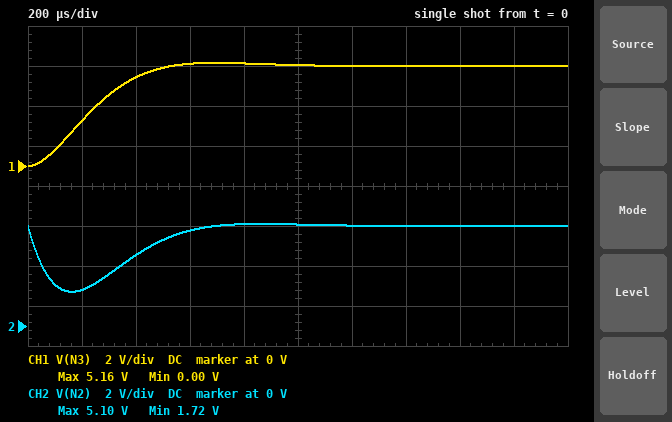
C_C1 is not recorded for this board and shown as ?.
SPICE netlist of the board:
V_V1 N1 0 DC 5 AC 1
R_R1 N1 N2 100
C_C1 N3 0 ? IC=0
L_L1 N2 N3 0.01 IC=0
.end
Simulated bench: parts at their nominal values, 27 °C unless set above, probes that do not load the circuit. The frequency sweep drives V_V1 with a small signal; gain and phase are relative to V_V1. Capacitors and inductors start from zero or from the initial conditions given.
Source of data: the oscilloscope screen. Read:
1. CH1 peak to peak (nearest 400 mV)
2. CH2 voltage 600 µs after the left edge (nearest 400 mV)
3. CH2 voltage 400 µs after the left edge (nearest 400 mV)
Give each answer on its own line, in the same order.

5.2 V
4.8 V
3.6 V
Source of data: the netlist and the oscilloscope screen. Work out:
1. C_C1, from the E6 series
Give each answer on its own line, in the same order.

2.2 µF
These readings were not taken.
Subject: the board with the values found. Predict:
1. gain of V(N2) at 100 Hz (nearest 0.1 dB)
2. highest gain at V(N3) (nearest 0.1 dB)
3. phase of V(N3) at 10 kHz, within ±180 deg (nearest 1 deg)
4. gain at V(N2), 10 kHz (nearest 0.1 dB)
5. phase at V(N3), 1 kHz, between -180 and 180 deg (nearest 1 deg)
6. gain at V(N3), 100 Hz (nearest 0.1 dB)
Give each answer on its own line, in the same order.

-0.1 dB
0 dB
-171 deg
-0.1 dB
-85 deg
0 dB
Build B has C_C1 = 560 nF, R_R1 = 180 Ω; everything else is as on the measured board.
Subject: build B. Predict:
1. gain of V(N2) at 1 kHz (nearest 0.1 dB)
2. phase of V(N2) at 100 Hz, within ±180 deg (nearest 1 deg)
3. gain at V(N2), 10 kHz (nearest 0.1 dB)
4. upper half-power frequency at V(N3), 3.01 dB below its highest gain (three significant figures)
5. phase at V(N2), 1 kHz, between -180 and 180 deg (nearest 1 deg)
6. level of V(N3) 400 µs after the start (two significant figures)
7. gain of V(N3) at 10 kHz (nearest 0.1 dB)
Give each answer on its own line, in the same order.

-2.2 dB
-4 deg
-0.4 dB
2.22 kHz
-39 deg
5.2 V
-26.9 dB
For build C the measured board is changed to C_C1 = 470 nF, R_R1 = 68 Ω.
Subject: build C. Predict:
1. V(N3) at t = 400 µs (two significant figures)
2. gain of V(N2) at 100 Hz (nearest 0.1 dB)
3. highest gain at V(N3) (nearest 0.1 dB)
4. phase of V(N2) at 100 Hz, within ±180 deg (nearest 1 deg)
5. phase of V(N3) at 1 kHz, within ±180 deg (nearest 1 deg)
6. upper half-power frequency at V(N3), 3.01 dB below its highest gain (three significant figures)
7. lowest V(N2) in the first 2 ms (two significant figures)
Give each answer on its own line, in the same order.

4.1 V
0 dB
6.9 dB
-1 deg
-14 deg
2.69 kHz
3.3 V
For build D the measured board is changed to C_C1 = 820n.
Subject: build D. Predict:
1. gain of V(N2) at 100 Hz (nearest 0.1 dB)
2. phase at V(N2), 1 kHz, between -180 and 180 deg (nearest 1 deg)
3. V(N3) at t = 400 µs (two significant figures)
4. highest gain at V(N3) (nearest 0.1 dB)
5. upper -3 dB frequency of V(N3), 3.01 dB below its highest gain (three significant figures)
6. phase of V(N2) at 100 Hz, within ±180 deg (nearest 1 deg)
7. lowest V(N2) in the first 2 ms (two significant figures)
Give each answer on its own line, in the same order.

0 dB
-37 deg
5.7 V
1.9 dB
2.08 kHz
-3 deg
2.4 V
